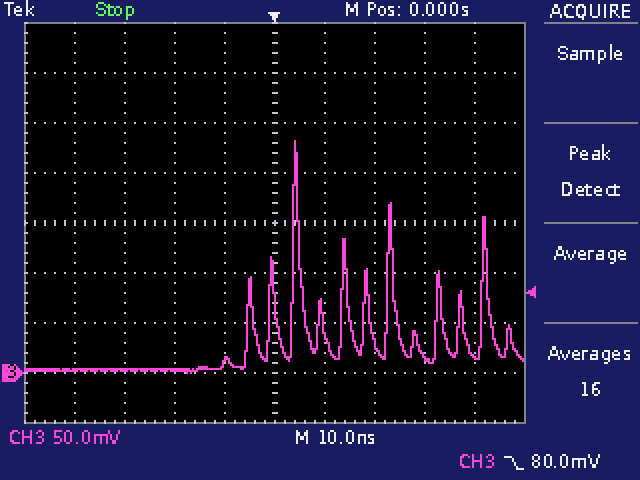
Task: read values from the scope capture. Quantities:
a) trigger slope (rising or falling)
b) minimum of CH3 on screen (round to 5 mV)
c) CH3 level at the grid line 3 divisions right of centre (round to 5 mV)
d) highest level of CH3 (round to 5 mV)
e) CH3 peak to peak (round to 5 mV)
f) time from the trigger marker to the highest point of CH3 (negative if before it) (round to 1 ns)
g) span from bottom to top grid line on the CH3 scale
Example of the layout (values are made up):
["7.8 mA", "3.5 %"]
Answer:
["falling", "0 mV", "15 mV", "230 mV", "230 mV", "+4 ns", "400 mV"]
